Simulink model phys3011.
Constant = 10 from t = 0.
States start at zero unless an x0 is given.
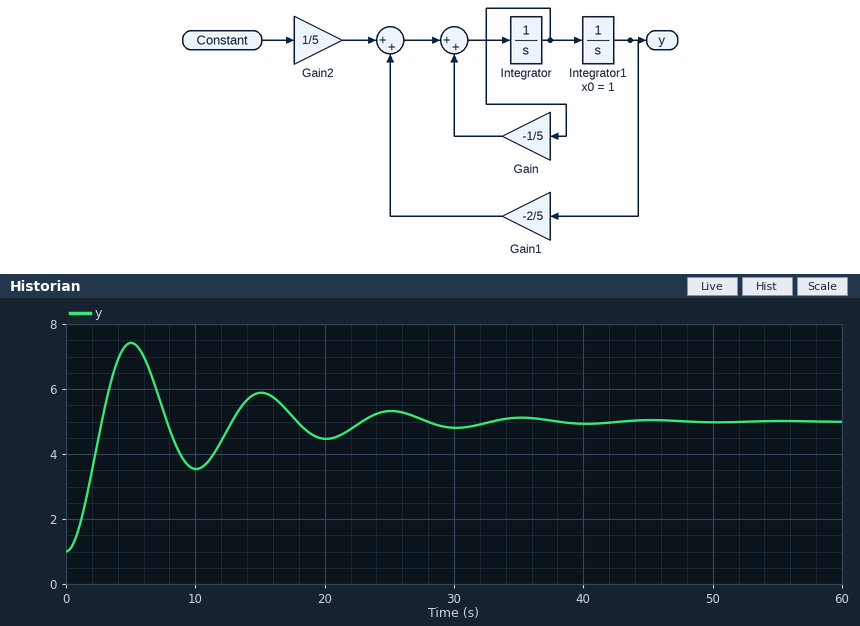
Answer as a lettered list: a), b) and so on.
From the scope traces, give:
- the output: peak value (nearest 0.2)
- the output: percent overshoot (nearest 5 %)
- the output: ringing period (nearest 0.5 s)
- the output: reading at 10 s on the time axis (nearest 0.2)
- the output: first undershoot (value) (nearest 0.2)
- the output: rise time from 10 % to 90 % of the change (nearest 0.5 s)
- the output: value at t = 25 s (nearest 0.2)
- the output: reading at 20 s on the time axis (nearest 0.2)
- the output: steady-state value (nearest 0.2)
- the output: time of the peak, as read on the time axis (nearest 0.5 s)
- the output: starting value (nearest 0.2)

a) 7.4
b) 60 %
c) 10.0 s
d) 3.6
e) 3.6
f) 2.0 s
g) 5.4
h) 4.4
i) 5.0
j) 5.0 s
k) 1.0
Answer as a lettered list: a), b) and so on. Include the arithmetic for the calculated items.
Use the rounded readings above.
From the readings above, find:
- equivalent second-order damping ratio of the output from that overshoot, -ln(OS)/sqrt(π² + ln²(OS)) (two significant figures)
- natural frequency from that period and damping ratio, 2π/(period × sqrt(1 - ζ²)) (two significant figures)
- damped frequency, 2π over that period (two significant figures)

a) ln(0.6) = -0.511; 0.511 / sqrt(9.870 + 0.261) = 0.16
b) 2π / (10 × sqrt(1 - 0.16²)) = 0.64 rad/s
c) 2π / 10 = 0.63 rad/s
